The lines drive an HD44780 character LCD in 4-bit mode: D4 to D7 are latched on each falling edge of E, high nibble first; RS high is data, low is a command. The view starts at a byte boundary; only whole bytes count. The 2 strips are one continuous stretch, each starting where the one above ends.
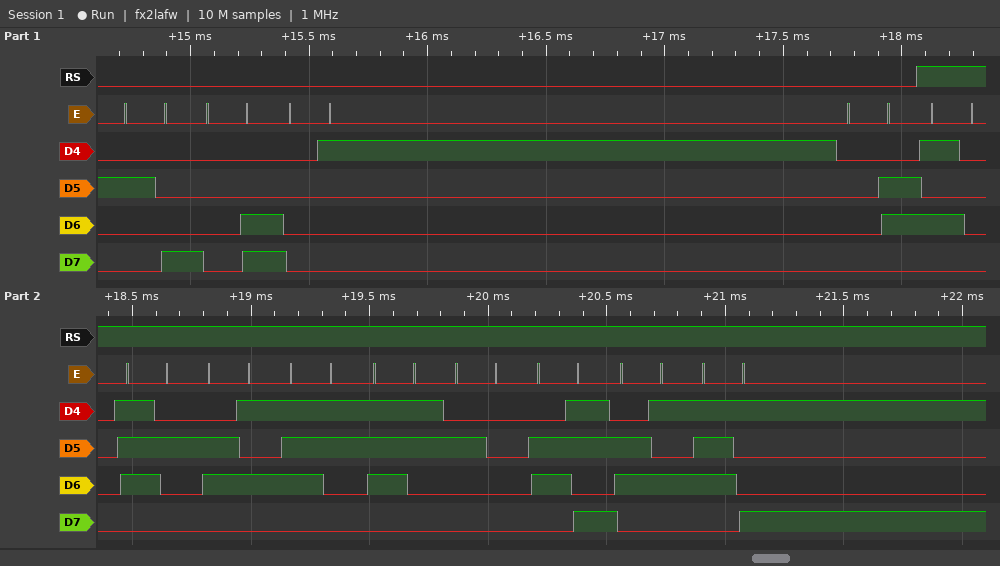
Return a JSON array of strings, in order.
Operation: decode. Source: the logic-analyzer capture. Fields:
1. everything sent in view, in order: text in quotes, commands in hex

["0x28 0x0C 0x01 0x06 \"Press key\""]
